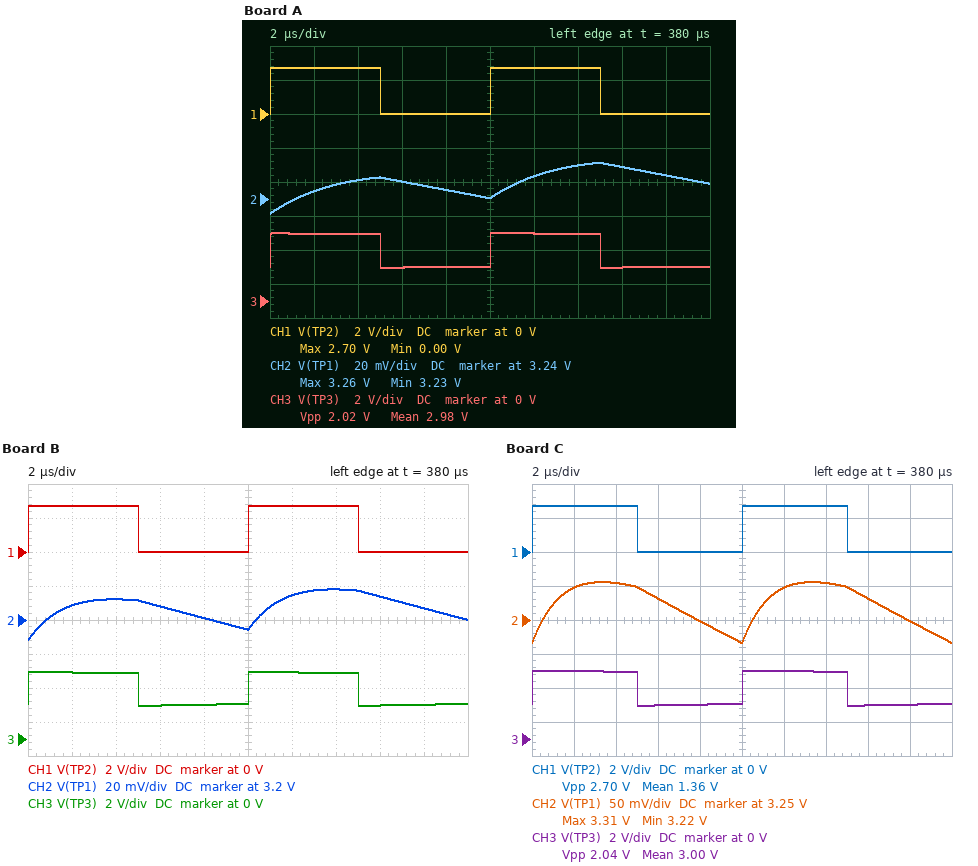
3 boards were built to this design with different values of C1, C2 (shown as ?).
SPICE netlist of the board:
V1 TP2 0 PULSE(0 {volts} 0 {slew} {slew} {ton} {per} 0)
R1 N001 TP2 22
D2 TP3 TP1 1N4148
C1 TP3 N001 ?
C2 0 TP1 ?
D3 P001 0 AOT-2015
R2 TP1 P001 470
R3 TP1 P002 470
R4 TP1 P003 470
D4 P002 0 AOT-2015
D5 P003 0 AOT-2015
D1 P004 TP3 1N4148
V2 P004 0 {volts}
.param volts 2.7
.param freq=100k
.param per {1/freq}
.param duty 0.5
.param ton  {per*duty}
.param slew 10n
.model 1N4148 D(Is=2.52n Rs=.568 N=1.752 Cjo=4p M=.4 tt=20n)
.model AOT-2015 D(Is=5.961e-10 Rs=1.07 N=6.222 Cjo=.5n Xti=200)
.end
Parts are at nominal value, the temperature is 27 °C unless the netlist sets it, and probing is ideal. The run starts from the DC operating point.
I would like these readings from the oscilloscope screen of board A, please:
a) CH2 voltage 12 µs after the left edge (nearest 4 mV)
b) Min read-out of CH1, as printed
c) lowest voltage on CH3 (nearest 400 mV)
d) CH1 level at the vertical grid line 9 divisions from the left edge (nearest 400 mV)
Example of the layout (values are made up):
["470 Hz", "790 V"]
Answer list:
["3.252 V", "0.00 V", "2.0 V", "0 V"]
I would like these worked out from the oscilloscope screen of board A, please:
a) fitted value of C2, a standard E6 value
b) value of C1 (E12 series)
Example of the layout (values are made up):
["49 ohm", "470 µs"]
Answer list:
["2.2 µF", "180 nF"]
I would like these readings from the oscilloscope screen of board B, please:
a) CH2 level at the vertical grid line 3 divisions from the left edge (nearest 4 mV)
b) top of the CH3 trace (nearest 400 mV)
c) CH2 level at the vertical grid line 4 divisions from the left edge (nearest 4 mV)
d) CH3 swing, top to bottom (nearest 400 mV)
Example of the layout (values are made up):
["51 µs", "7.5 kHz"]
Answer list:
["3.208 V", "4.0 V", "3.200 V", "2.0 V"]
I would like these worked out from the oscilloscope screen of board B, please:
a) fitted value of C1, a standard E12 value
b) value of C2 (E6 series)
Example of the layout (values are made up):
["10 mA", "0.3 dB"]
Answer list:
["82 nF", "1.5 µF"]
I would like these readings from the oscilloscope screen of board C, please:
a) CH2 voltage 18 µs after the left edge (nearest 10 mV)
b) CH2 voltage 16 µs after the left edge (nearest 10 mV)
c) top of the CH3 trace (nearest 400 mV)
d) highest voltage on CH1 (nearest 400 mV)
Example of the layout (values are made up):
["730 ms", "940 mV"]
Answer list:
["3.25 V", "3.28 V", "4.0 V", "2.8 V"]
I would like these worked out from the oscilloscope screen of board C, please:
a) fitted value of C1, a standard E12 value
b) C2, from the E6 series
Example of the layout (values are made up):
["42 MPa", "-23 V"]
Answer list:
["82 nF", "330 nF"]
